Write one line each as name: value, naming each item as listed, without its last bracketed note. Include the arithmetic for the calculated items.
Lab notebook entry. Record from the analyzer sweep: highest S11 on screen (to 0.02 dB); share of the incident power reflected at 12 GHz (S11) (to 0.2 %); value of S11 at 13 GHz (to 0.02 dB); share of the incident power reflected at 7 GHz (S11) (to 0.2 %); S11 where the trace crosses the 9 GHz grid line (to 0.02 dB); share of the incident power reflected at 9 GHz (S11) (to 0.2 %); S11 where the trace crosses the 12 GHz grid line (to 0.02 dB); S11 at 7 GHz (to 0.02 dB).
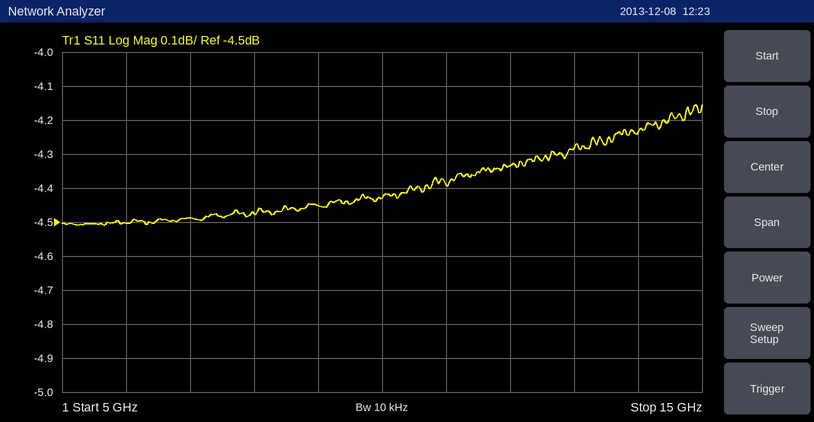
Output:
highest S11 on screen: -4.16 dB
share of the incident power reflected at 12 GHz (S11): 10^(-4.34/10) ≈ 36.8 %
value of S11 at 13 GHz: -4.28 dB
share of the incident power reflected at 7 GHz (S11): 10^(-4.48/10) ≈ 35.6 %
S11 where the trace crosses the 9 GHz grid line: -4.46 dB
share of the incident power reflected at 9 GHz (S11): 10^(-4.46/10) ≈ 35.8 %
S11 where the trace crosses the 12 GHz grid line: -4.34 dB
S11 at 7 GHz: -4.48 dB
